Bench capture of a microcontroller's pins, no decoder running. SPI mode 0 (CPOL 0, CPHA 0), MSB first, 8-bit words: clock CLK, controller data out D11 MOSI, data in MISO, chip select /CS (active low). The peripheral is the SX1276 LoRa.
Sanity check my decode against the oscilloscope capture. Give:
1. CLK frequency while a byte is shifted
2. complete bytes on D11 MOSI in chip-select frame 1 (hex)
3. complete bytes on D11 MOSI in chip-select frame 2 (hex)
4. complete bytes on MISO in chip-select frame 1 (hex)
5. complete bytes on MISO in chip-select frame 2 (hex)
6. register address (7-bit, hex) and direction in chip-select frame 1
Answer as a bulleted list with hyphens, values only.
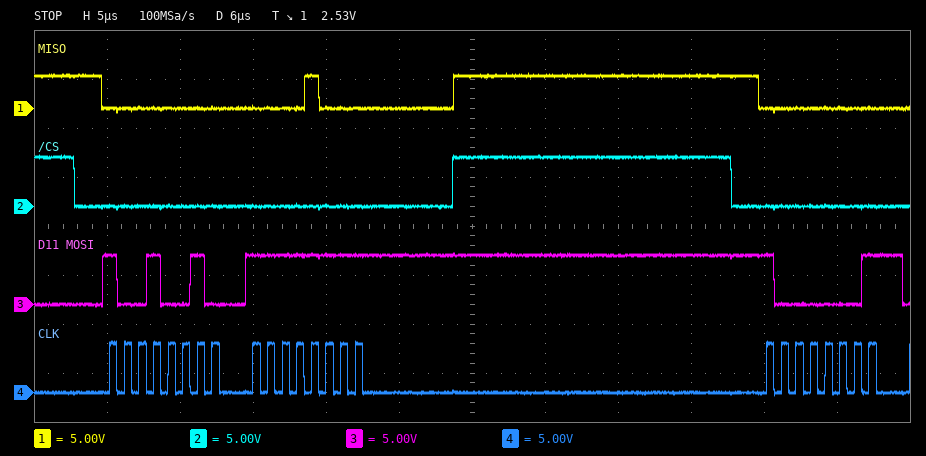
- 1 MHz
- 92 FF
- 81
- 00 08
- 00
- 0x12 write
